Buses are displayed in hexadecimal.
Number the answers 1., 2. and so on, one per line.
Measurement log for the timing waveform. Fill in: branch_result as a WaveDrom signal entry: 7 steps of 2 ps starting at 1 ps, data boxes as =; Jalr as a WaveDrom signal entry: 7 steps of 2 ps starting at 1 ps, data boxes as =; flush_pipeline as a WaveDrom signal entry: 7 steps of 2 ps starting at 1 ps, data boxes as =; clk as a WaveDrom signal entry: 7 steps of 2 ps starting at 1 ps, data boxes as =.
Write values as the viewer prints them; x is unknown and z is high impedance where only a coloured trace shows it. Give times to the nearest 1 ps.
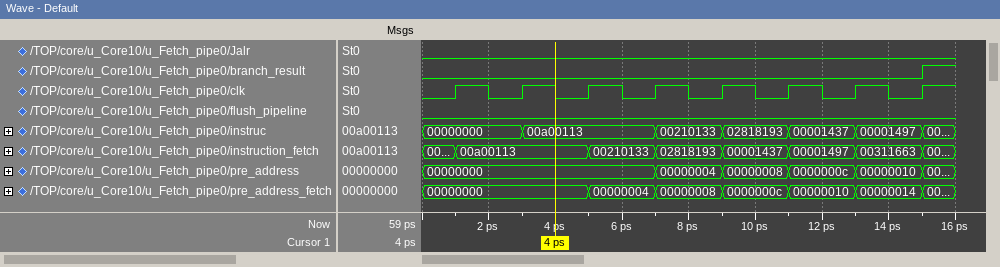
1. {name: 'branch_result', wave: '0......'}
2. {name: 'Jalr', wave: '0......'}
3. {name: 'flush_pipeline', wave: '0......'}
4. {name: 'clk', wave: 'p......'}
